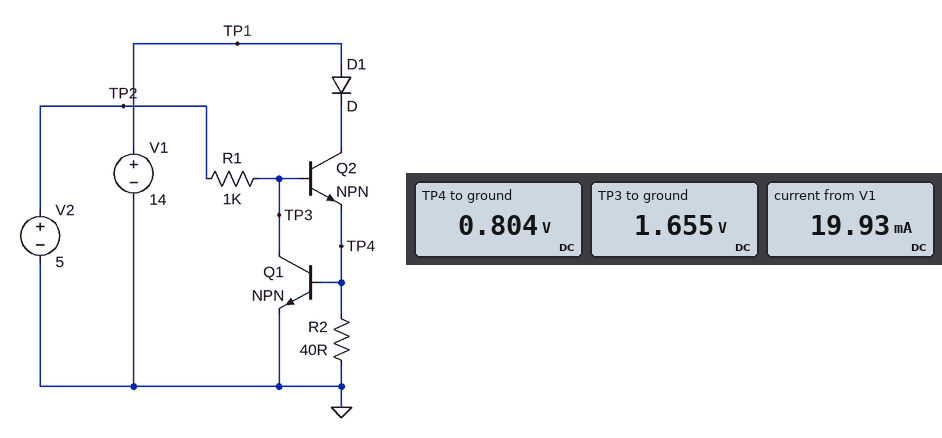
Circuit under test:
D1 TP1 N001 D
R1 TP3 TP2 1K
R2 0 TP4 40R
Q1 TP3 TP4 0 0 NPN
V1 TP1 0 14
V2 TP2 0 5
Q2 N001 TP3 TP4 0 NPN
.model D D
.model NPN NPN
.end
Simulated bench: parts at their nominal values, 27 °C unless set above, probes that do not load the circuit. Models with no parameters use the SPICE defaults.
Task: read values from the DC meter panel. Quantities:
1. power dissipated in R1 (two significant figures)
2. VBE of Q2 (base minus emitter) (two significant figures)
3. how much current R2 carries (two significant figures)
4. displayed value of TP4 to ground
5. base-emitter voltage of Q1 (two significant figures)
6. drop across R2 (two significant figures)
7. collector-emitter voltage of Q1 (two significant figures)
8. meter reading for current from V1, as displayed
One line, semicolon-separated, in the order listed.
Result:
11 mW; 850 mV; 20 mA; 0.804 V; 800 mV; 800 mV; 1.7 V; 19.93 mA
